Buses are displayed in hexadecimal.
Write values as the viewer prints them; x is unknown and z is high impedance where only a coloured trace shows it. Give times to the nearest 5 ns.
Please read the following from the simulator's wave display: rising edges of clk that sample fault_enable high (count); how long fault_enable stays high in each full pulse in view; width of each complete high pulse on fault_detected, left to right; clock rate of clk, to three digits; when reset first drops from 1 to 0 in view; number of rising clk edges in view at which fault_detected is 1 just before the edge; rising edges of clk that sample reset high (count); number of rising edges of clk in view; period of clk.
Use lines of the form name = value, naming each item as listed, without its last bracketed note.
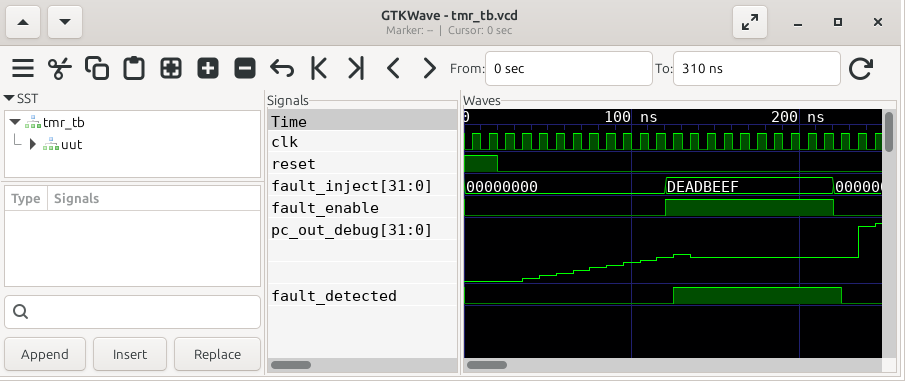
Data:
rising edges of clk that sample fault_enable high = 10
how long fault_enable stays high in each full pulse in view = 100 ns
width of each complete high pulse on fault_detected, left to right = 100 ns
clock rate of clk, to three digits = 100 MHz
when reset first drops from 1 to 0 in view = 20 ns
number of rising clk edges in view at which fault_detected is 1 just before the edge = 10
rising edges of clk that sample reset high = 2
number of rising edges of clk in view = 25
period of clk = 10 ns
